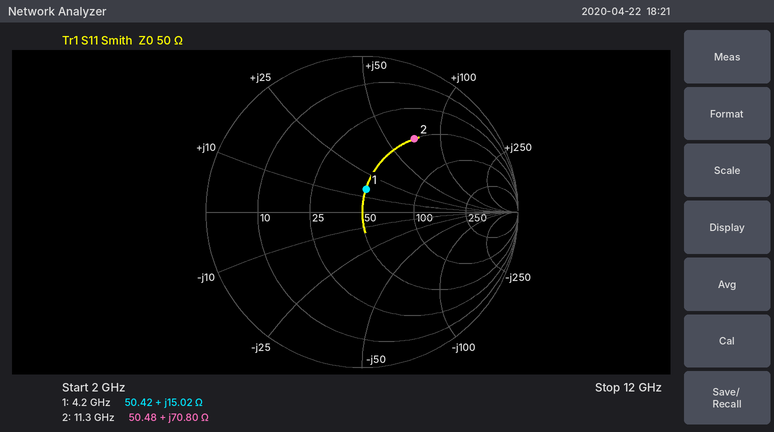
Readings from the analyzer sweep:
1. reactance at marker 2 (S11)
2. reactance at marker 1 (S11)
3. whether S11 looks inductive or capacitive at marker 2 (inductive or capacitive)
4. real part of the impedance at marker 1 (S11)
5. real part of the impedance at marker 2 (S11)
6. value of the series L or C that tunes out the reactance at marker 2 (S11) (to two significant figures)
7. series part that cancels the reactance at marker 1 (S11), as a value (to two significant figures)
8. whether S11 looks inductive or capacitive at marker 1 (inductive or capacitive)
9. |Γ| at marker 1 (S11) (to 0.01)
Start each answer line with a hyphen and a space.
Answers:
- +70.80 Ω
- +15.02 Ω
- inductive
- 50.42 Ω
- 50.48 Ω
- 200 fF
- 2.5 pF
- inductive
- 0.15
